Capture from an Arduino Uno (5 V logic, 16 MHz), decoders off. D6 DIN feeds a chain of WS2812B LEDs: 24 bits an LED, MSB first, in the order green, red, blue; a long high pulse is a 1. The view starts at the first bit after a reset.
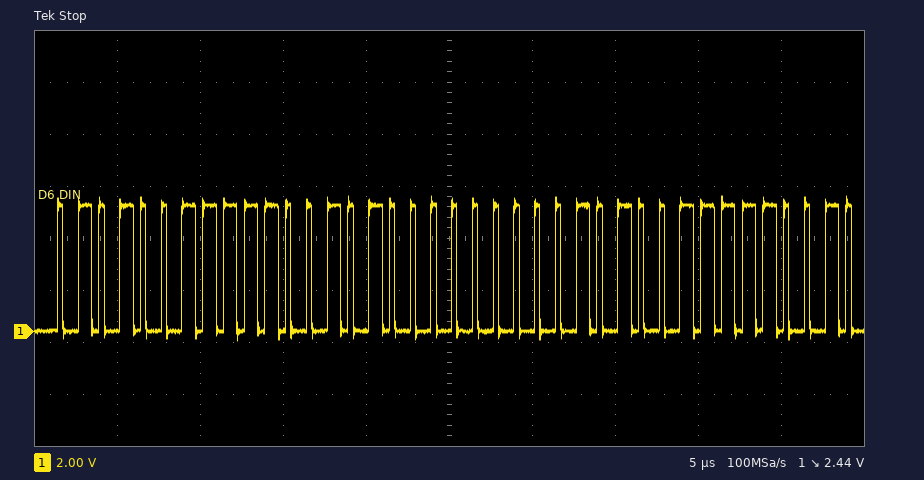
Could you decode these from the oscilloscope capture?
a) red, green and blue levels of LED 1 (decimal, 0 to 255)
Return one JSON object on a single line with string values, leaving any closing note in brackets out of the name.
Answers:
{"red, green and blue levels of LED 1": "229, 83, 0"}
